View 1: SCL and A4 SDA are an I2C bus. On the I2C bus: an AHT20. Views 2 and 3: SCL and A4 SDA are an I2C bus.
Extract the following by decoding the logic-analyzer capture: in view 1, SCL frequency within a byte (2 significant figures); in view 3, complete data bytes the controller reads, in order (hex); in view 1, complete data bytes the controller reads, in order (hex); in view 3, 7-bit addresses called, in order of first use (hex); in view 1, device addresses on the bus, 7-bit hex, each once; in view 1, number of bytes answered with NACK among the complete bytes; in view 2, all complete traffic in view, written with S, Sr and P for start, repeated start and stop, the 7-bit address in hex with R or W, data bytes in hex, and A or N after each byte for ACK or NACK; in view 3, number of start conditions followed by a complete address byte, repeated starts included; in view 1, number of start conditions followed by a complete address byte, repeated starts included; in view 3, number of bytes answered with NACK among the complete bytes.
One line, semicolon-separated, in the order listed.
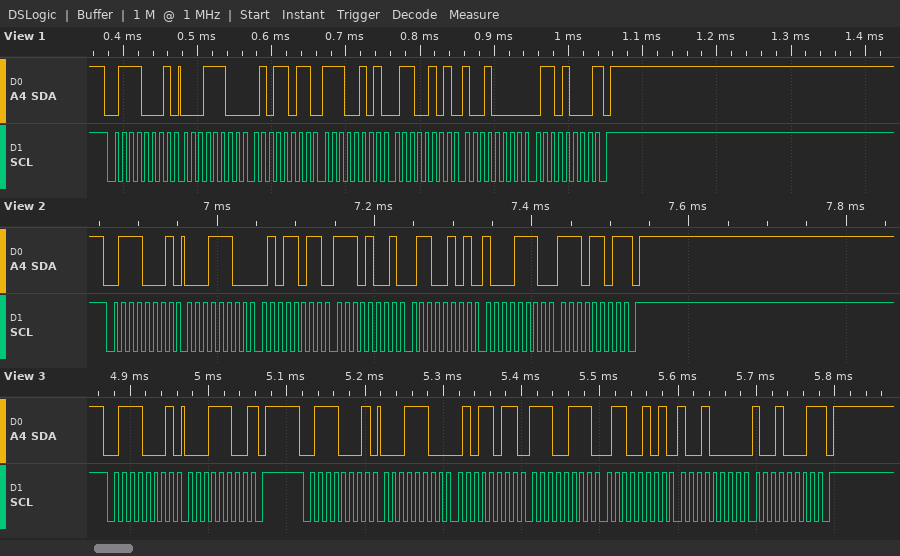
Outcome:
100 kHz; 1C 1C 5B E7 65 90 91; 1C 5B E5 65 90 68; 0x38; 0x38; 1; S 38R A 1C A 5B A E9 A 65 A 8E A ED N P; 2; 1; 2
